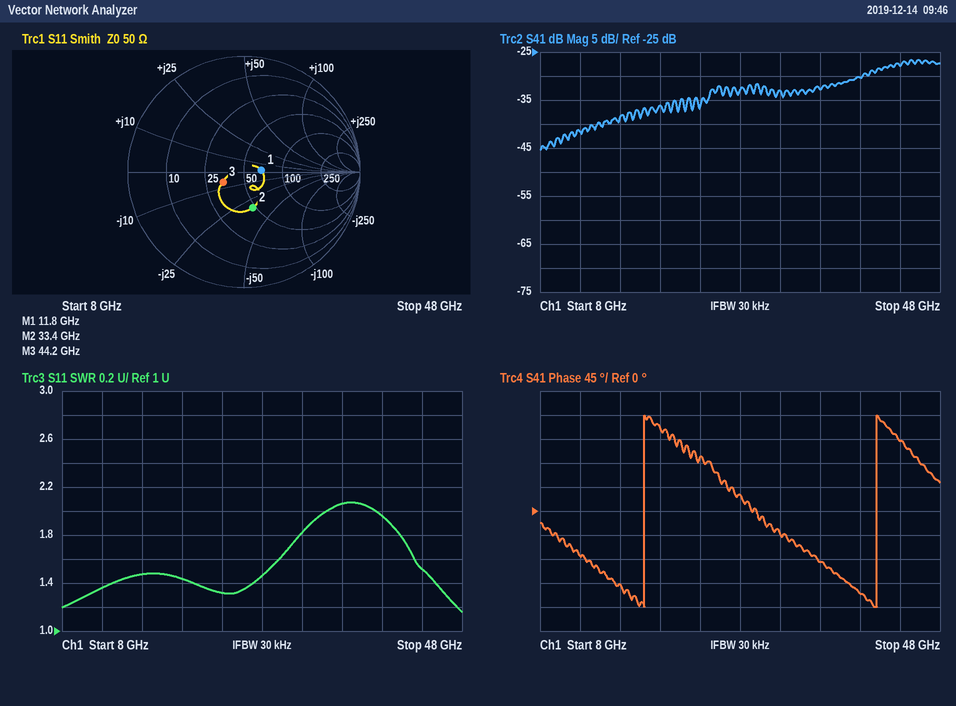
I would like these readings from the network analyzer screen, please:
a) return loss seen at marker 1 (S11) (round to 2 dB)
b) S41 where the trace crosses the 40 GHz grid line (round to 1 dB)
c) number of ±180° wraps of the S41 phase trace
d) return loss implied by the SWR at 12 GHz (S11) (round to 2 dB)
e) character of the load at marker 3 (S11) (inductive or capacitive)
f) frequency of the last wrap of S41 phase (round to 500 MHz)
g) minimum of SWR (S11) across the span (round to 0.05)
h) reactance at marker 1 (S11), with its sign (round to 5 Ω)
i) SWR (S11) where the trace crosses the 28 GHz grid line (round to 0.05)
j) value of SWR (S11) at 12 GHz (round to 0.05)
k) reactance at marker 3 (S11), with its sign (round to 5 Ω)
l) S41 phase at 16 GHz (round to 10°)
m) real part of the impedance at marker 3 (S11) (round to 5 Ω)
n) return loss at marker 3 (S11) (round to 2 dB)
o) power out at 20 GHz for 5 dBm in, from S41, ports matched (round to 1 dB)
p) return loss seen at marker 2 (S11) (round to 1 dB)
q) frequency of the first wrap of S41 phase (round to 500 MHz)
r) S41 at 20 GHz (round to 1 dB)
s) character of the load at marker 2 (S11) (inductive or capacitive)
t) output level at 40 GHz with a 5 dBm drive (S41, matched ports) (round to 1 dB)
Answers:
16 dB
-30 dB
2
16 dB
capacitive
41.5 GHz
1.15
0 Ω
1.45
1.35
-5 Ω
-140°
35 Ω
14 dB
-31 dBm
10 dB
18.5 GHz
-36 dB
capacitive
-25 dBm
